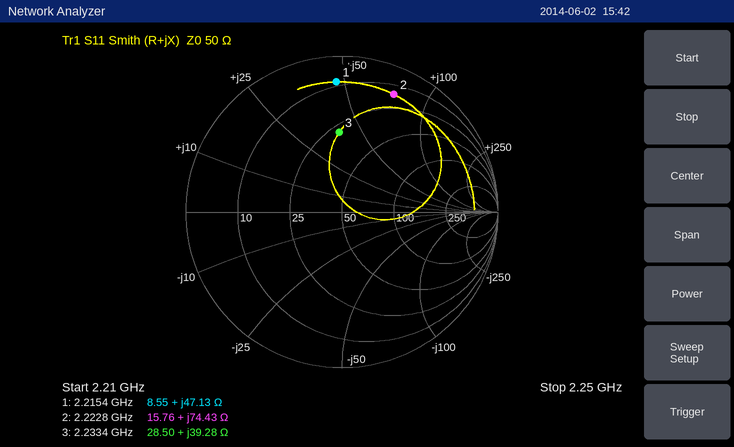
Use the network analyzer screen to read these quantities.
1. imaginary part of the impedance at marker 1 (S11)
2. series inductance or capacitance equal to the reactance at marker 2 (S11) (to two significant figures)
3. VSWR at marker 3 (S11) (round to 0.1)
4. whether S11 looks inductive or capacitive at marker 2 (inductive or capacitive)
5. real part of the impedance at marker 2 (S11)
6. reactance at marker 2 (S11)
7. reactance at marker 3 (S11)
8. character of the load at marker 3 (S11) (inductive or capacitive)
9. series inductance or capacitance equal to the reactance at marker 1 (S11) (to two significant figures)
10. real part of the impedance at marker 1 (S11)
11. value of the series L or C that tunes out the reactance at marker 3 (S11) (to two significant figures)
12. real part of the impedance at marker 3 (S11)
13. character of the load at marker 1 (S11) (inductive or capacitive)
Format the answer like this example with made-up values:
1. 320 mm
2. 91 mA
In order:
1. +47.13 Ω
2. 5.3 nH
3. 3.1
4. inductive
5. 15.76 Ω
6. +74.43 Ω
7. +39.28 Ω
8. inductive
9. 3.4 nH
10. 8.55 Ω
11. 1.8 pF
12. 28.50 Ω
13. inductive
